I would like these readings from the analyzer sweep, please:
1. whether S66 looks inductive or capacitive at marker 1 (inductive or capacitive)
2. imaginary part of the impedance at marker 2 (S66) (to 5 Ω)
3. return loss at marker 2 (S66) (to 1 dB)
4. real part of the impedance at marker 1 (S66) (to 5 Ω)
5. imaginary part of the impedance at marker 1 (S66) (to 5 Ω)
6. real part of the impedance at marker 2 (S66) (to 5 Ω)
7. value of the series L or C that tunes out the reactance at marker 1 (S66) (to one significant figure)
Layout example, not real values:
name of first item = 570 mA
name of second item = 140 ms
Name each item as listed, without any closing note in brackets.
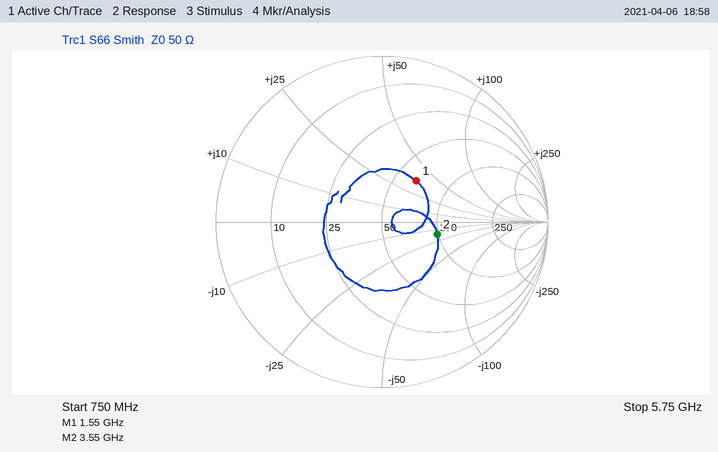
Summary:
whether S66 looks inductive or capacitive at marker 1 = inductive
imaginary part of the impedance at marker 2 (S66) = -15 Ω
return loss at marker 2 (S66) = 9 dB
real part of the impedance at marker 1 (S66) = 65 Ω
imaginary part of the impedance at marker 1 (S66) = +35 Ω
real part of the impedance at marker 2 (S66) = 100 Ω
value of the series L or C that tunes out the reactance at marker 1 (S66) = 3 pF
